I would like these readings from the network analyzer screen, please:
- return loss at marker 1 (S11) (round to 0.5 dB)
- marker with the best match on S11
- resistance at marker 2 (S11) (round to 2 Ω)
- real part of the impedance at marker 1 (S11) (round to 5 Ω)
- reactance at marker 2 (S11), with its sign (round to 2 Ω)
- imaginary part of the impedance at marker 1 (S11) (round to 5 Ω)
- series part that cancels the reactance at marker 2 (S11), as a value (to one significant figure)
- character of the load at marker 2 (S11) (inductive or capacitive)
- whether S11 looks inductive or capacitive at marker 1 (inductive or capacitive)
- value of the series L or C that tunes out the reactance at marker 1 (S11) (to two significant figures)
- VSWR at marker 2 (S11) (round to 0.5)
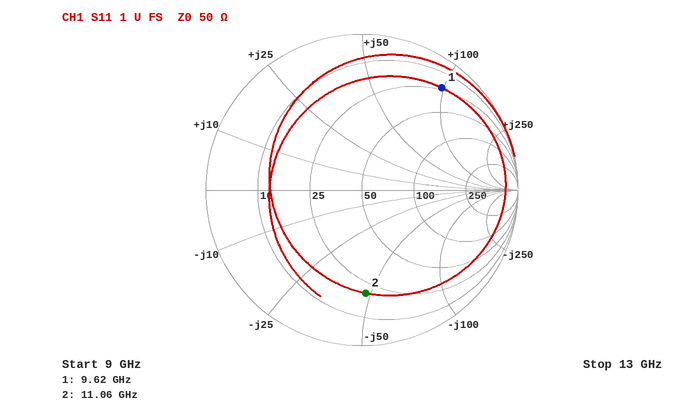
1.5 dB
marker 2
20 Ω
25 Ω
-48 Ω
+100 Ω
700 pH
capacitive
inductive
170 fF
5.0
